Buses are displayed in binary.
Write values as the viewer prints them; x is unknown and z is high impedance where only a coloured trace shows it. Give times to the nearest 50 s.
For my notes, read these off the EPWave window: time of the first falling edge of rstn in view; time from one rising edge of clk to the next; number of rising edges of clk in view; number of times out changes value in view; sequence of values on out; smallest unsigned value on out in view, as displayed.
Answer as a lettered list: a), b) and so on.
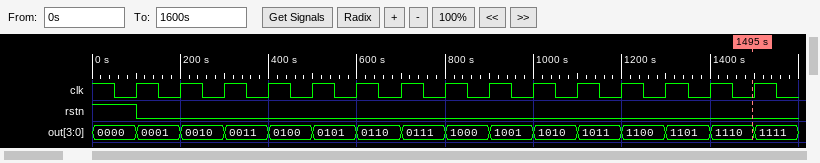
a) 100 s
b) 100 s
c) 15
d) 15
e) 0000, 0001, 0010, 0011, 0100, 0101, 0110, 0111, 1000, 1001, 1010, 1011, 1100, 1101, 1110, 1111
f) 0000
